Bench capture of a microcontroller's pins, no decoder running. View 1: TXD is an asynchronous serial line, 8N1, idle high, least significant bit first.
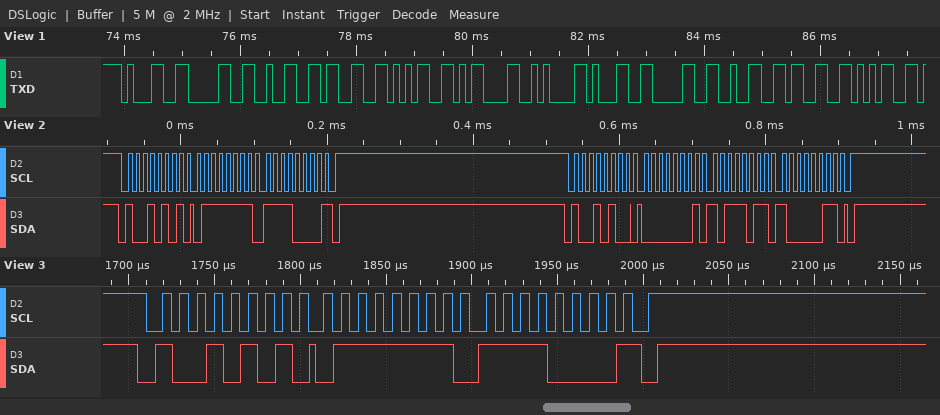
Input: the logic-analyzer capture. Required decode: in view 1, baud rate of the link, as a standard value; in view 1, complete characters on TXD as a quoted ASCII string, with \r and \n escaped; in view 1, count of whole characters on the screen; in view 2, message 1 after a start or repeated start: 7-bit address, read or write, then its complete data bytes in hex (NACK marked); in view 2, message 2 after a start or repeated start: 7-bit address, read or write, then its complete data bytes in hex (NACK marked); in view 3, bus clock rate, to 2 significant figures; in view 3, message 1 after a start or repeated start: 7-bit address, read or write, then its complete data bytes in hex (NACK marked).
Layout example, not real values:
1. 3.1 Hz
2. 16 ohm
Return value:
1. 9600 baud
2. "10235\r\n10235"
3. 12
4. 0x4A read: 7F F0 NACK
5. 0x4A write: 01 BB 83
6. 100 kHz
7. 0x4A read: 7F F0 NACK
